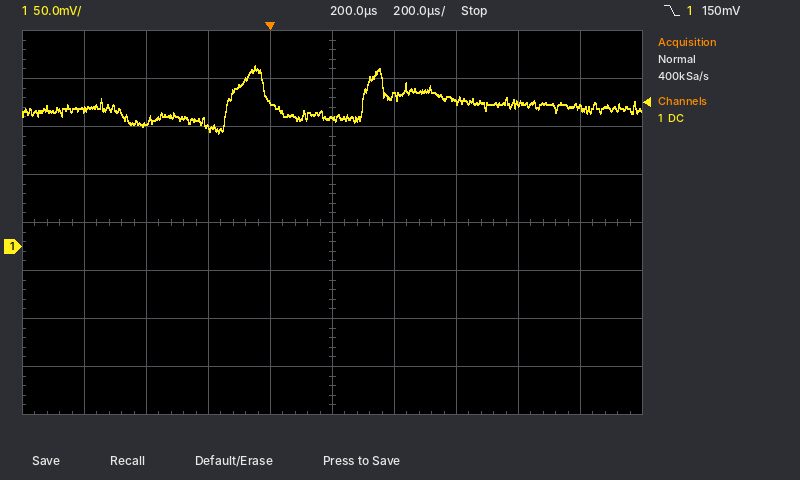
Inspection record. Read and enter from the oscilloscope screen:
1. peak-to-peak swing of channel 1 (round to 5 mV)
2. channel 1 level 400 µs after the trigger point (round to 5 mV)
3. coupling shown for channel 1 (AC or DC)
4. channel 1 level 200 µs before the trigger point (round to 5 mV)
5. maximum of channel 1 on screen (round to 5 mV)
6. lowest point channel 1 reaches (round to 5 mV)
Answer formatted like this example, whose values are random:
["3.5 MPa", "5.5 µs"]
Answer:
["70 mV", "155 mV", "DC", "125 mV", "190 mV", "120 mV"]
